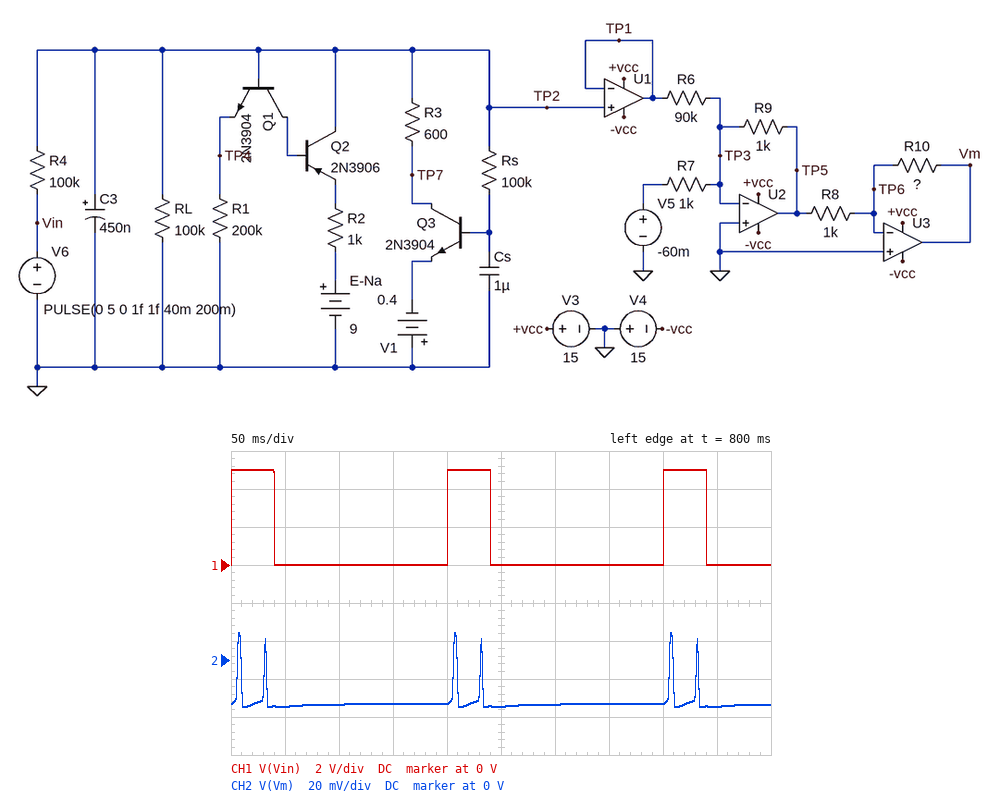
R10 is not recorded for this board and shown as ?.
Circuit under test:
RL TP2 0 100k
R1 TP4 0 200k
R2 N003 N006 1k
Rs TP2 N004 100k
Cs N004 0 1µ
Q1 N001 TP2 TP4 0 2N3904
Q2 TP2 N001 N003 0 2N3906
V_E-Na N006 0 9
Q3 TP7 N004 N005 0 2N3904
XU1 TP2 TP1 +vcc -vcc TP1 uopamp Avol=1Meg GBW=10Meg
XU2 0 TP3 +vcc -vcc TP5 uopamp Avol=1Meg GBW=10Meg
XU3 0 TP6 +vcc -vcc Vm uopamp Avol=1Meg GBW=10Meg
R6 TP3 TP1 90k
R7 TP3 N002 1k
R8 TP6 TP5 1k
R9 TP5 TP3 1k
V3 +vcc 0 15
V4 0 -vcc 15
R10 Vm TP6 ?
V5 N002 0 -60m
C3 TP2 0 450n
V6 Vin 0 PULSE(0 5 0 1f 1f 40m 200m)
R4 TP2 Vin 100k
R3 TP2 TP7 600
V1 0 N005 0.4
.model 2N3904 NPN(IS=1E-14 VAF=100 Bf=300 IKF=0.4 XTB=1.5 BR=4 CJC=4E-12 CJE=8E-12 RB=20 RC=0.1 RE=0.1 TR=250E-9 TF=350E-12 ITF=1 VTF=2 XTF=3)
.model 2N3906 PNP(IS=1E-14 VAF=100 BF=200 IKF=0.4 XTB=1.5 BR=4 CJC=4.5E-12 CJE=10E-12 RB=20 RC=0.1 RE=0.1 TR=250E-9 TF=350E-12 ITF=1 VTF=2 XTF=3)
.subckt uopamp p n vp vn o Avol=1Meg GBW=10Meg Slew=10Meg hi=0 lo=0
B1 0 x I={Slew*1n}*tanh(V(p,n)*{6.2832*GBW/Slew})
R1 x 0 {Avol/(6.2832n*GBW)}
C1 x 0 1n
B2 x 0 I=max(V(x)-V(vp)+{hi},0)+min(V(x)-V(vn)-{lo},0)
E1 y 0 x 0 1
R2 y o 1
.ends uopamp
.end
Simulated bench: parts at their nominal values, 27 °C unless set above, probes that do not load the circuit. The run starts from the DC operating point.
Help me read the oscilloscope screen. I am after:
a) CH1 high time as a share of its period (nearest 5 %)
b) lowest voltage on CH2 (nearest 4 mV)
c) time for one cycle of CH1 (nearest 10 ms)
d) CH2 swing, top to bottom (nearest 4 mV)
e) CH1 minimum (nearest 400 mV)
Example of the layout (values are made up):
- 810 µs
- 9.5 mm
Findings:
- 20 %
- -24 mV
- 200 ms
- 40 mV
- 0 V
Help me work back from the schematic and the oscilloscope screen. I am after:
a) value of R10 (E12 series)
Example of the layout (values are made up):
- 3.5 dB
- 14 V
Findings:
- 390 Ω
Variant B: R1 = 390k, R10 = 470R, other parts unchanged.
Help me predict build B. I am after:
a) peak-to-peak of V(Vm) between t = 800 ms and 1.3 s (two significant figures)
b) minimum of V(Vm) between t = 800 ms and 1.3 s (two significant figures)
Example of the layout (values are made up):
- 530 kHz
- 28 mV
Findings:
- 47 mV
- -30 mV
